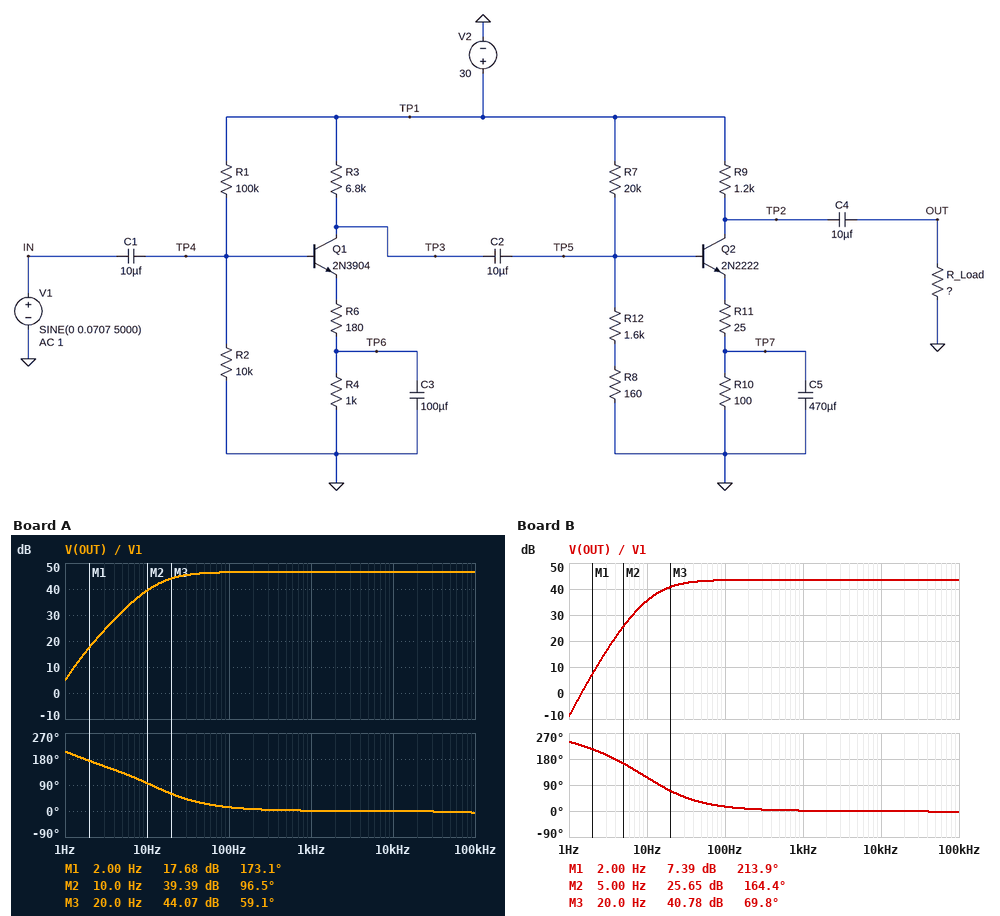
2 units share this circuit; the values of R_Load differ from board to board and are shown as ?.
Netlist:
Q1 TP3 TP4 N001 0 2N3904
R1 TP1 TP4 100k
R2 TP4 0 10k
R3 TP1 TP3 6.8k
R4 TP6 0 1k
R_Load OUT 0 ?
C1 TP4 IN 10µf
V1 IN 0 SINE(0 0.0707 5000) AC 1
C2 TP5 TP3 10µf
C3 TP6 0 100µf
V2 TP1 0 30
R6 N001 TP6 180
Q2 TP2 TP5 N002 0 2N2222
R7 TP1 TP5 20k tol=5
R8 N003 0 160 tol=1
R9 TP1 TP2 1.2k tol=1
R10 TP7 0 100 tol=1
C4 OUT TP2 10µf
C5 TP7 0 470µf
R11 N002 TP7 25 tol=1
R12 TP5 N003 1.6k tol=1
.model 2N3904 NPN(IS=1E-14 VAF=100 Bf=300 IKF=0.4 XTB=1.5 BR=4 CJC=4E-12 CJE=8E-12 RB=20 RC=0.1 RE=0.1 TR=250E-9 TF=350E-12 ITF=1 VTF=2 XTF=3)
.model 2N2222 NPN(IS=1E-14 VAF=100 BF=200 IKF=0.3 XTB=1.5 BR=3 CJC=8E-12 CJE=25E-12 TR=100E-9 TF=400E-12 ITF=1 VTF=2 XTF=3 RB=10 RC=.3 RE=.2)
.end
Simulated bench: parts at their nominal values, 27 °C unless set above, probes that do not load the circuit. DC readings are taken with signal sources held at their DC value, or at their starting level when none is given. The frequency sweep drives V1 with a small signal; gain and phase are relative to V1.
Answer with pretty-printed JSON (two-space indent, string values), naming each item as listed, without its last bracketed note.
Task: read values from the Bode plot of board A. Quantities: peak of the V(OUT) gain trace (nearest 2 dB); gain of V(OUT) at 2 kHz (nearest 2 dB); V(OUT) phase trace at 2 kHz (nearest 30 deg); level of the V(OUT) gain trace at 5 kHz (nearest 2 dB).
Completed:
{
  "peak of the V(OUT) gain trace": "46 dB",
  "gain of V(OUT) at 2 kHz": "46 dB",
  "V(OUT) phase trace at 2 kHz": "0 deg",
  "level of the V(OUT) gain trace at 5 kHz": "46 dB"
}
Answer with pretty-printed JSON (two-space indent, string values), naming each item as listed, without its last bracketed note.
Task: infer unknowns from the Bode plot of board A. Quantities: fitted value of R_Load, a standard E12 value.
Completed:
{
  "fitted value of R_Load, a standard E12 value": "15 kΩ"
}
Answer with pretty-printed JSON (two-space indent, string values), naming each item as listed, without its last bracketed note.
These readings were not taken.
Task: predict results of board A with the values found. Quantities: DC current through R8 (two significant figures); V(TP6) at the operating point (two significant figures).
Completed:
{
  "DC current through R8": "1.3 mA",
  "V(TP6) at the operating point": "1.7 V"
}
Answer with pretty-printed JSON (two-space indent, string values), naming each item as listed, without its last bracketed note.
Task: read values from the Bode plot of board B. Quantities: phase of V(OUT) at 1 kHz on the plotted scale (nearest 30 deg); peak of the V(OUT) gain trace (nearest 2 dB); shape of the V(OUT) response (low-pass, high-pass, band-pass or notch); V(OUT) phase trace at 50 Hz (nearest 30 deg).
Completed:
{
  "phase of V(OUT) at 1 kHz on the plotted scale": "0 deg",
  "peak of the V(OUT) gain trace": "44 dB",
  "shape of the V(OUT) response": "high-pass",
  "V(OUT) phase trace at 50 Hz": "30 deg"
}
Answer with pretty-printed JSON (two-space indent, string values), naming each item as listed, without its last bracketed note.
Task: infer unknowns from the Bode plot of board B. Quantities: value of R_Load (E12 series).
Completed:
{
  "value of R_Load": "2.2 kΩ"
}
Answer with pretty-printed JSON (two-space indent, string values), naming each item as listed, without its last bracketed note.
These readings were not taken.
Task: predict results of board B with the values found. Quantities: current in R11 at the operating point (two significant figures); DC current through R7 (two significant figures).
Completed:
{
  "current in R11 at the operating point": "13 mA",
  "DC current through R7": "1.4 mA"
}
